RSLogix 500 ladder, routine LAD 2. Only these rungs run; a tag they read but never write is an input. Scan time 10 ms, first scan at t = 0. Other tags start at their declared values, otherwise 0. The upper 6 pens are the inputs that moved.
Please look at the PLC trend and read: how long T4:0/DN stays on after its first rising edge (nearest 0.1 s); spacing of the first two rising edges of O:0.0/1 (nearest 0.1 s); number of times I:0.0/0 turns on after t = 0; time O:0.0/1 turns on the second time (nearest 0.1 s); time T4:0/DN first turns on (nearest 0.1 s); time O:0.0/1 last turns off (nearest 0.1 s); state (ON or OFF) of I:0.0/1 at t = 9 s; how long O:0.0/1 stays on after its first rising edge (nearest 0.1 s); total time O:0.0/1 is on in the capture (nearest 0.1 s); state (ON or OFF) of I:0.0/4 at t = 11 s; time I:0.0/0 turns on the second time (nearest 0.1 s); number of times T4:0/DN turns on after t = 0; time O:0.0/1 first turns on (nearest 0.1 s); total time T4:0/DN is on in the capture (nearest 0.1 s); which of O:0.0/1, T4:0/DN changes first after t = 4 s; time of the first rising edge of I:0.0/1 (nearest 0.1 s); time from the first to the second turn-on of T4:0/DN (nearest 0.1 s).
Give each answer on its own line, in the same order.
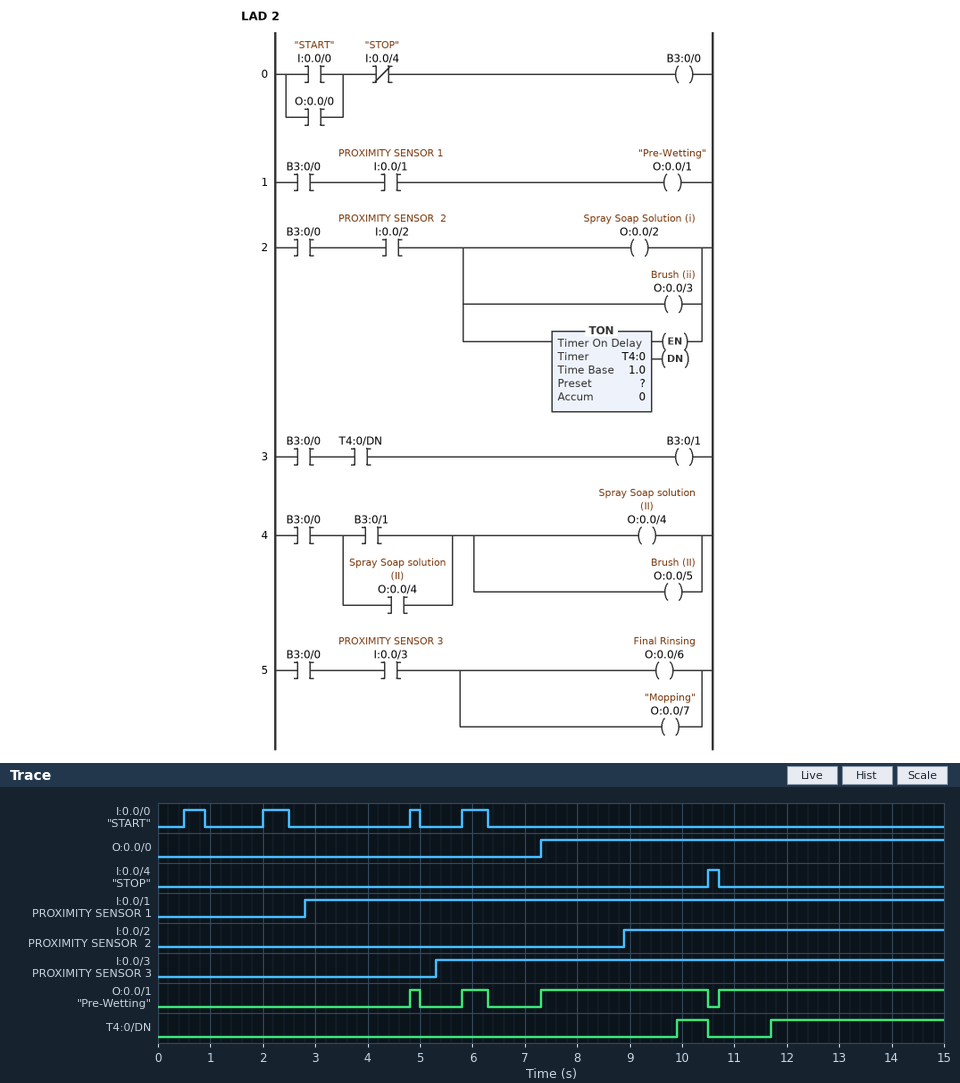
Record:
0.6 s
1.0 s
4
5.8 s
9.9 s
10.5 s
ON
0.2 s
8.2 s
OFF
2.0 s
2
4.8 s
3.9 s
O:0.0/1
2.8 s
1.8 s
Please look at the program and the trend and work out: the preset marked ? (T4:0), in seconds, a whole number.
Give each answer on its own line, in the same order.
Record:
1 s
